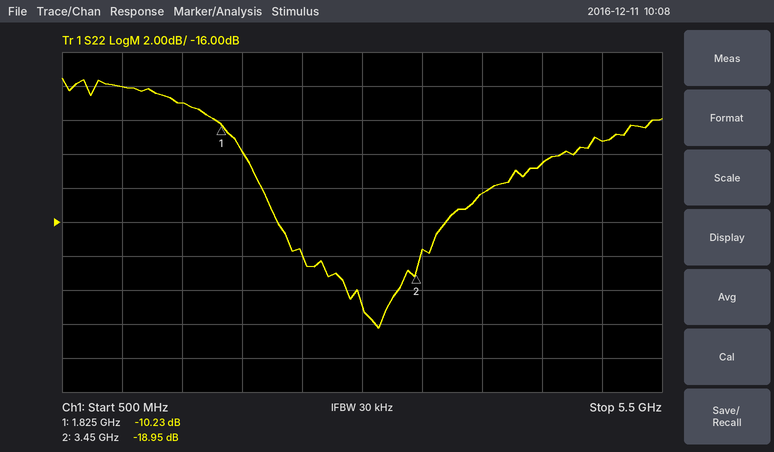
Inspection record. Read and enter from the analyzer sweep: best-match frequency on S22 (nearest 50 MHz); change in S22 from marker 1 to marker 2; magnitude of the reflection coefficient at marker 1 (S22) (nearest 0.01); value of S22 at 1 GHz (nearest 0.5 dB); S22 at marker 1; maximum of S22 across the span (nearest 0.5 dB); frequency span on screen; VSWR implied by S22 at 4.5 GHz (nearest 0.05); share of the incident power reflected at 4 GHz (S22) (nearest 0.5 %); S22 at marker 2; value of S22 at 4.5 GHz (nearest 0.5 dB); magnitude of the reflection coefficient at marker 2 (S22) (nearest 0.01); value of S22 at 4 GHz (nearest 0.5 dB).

3.15 GHz
-8.72 dB
0.31
-8.0 dB
-10.23 dB
-7.5 dB
5 GHz
1.60
3.5 %
-18.95 dB
-12.5 dB
0.11
-14.5 dB
